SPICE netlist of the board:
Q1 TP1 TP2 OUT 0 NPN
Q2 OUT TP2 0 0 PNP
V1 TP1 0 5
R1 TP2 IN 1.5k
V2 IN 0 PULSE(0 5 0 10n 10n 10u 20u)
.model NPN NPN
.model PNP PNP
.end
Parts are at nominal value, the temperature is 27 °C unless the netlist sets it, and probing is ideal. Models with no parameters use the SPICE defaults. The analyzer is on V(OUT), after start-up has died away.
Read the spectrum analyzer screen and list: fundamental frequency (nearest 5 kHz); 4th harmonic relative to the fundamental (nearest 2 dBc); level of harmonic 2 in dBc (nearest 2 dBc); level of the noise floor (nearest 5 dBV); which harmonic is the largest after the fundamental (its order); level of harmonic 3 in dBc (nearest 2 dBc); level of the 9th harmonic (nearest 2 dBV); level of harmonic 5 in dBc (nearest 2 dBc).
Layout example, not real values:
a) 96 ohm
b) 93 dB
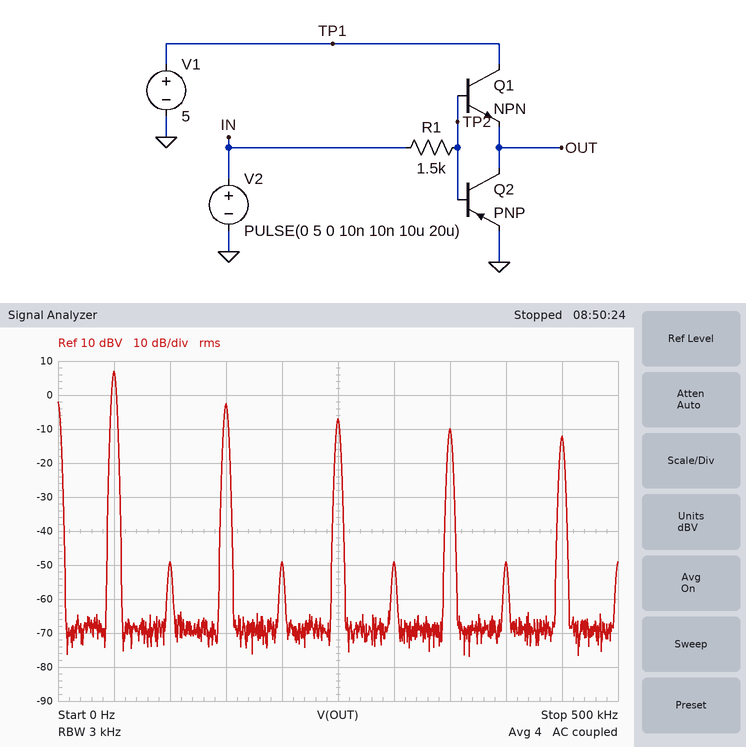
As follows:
a) 50 kHz
b) -56 dBc
c) -56 dBc
d) -70 dBV
e) 3
f) -10 dBc
g) -12 dBV
h) -14 dBc
